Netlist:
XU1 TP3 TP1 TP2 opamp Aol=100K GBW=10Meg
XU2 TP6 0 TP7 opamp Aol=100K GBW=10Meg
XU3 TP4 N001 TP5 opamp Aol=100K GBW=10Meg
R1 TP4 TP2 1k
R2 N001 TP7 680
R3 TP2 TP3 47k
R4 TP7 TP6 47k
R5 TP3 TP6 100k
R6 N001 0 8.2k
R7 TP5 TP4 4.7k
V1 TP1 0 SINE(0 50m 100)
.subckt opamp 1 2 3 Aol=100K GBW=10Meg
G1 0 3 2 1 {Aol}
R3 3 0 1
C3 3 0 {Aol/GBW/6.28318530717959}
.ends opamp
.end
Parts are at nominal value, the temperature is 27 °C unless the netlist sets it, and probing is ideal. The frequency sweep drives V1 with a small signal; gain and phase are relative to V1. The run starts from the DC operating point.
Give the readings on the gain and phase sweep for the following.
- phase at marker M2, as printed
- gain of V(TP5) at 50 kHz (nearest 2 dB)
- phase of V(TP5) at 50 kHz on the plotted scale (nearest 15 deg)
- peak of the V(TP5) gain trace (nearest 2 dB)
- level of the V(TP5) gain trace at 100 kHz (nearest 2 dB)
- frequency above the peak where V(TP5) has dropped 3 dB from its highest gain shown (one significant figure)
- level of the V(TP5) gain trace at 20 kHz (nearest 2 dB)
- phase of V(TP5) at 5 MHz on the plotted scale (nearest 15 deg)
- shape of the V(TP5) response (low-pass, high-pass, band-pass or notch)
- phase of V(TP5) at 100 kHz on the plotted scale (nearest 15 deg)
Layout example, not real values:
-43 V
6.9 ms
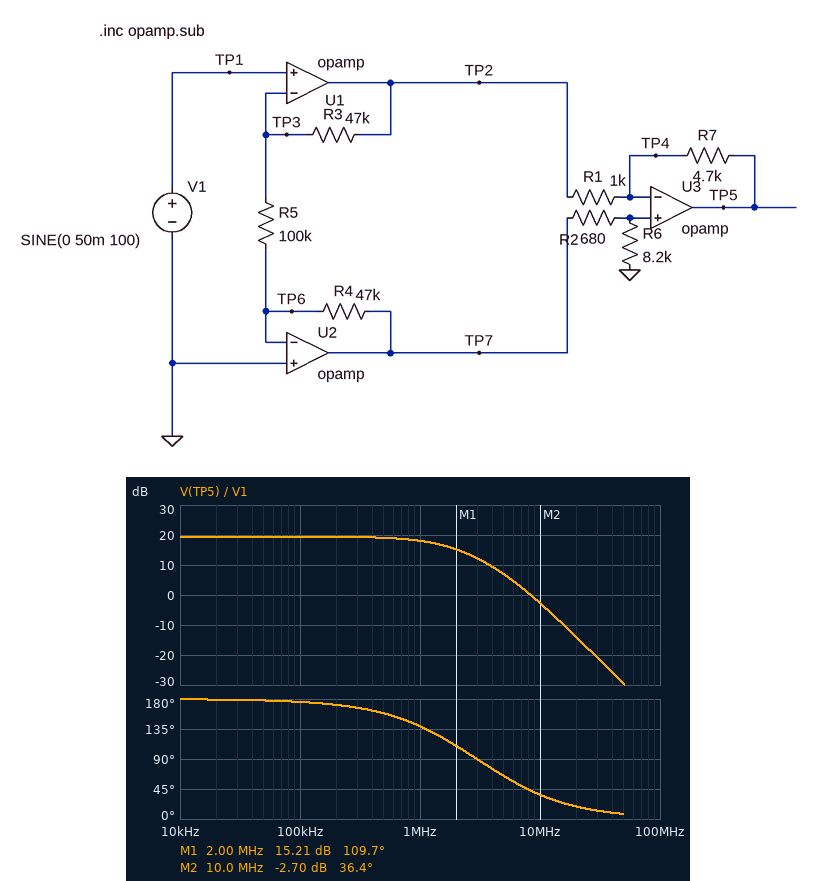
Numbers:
36.4 deg
20 dB
180 deg
20 dB
20 dB
2 MHz
20 dB
60 deg
low-pass
180 deg
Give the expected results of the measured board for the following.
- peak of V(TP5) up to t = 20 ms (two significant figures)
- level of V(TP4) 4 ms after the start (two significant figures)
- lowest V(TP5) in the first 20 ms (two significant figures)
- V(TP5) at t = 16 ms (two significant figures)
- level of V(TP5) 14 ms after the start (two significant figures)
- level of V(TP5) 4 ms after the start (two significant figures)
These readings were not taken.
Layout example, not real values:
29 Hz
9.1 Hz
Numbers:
470 mV
-13 mV
-470 mV
280 mV
-280 mV
-280 mV
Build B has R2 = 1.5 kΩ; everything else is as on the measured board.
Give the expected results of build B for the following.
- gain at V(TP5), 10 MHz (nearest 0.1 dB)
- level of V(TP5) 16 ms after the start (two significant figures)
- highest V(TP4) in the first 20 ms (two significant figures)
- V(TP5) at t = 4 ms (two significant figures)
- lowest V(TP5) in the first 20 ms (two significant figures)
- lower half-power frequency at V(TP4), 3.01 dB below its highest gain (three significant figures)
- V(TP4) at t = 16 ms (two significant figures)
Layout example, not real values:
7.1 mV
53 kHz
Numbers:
-2.8 dB
270 mV
20 mV
-270 mV
-460 mV
979 kHz
12 mV
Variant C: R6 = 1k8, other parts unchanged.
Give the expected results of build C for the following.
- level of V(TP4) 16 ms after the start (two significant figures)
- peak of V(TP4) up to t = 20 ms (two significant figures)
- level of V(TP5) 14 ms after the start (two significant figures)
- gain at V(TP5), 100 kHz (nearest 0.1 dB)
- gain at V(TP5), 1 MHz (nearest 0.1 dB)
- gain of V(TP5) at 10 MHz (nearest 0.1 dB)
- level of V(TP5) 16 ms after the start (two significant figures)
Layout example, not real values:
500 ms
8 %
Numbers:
10 mV
17 mV
-260 mV
18.9 dB
17.6 dB
-3.0 dB
260 mV
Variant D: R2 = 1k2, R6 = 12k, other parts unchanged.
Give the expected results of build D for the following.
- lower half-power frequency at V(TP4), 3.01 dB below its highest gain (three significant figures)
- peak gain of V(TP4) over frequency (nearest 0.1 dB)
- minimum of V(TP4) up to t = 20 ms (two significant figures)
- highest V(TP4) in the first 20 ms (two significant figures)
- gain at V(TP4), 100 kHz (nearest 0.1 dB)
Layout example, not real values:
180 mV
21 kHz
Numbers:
949 kHz
0.1 dB
-21 mV
21 mV
-7.3 dB
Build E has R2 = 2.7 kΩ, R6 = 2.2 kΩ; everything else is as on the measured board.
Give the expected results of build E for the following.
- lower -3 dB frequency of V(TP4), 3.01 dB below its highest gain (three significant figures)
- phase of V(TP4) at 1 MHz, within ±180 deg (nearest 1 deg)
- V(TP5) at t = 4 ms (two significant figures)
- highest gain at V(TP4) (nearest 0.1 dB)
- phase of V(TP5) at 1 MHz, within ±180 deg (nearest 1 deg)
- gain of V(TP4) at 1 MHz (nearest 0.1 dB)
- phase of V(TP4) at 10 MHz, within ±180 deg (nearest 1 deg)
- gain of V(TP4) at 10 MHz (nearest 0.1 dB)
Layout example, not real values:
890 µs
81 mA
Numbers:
1.11 MHz
67 deg
-240 mV
-0.3 dB
140 deg
-3.9 dB
-44 deg
-3.7 dB
